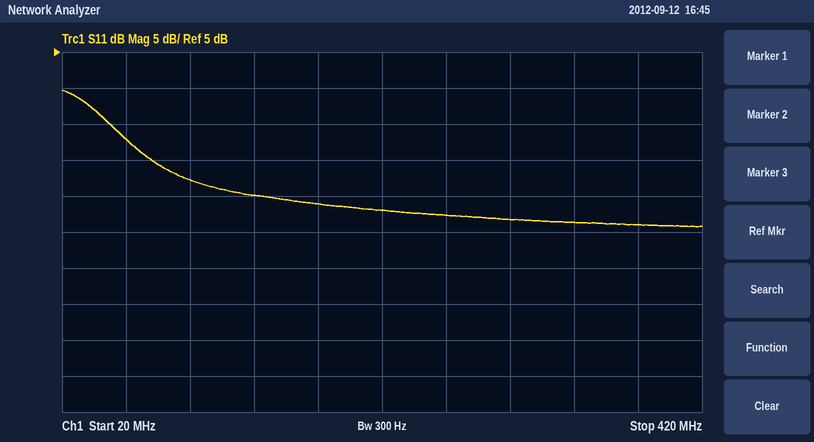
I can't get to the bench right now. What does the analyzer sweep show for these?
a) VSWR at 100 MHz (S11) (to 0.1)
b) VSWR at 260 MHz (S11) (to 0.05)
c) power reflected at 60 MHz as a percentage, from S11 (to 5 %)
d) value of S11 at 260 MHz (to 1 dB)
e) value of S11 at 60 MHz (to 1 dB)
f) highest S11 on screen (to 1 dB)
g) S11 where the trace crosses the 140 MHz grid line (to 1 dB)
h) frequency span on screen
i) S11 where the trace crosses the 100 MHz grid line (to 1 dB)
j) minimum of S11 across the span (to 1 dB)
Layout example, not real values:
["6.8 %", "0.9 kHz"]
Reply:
["1.6", "1.30", "20 %", "-18 dB", "-7 dB", "0 dB", "-15 dB", "400 MHz", "-13 dB", "-19 dB"]
